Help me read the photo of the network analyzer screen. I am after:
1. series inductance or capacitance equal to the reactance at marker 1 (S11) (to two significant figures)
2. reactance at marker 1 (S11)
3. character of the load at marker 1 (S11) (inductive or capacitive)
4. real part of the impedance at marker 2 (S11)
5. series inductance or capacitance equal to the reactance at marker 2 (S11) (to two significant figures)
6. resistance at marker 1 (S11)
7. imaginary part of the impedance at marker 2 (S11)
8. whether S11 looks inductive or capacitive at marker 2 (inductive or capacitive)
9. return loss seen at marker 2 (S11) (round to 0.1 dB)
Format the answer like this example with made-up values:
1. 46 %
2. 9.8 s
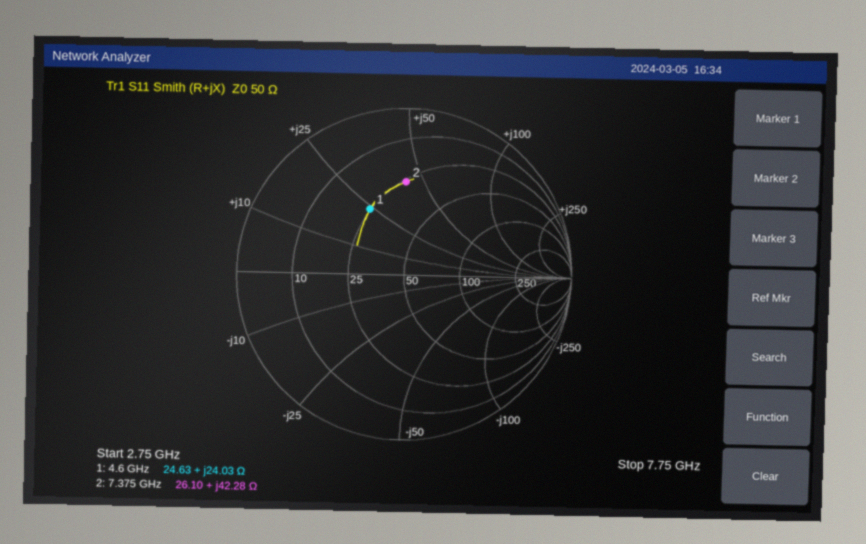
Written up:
1. 830 pH
2. +24.03 Ω
3. inductive
4. 26.10 Ω
5. 910 pH
6. 24.63 Ω
7. +42.28 Ω
8. inductive
9. 5.1 dB
